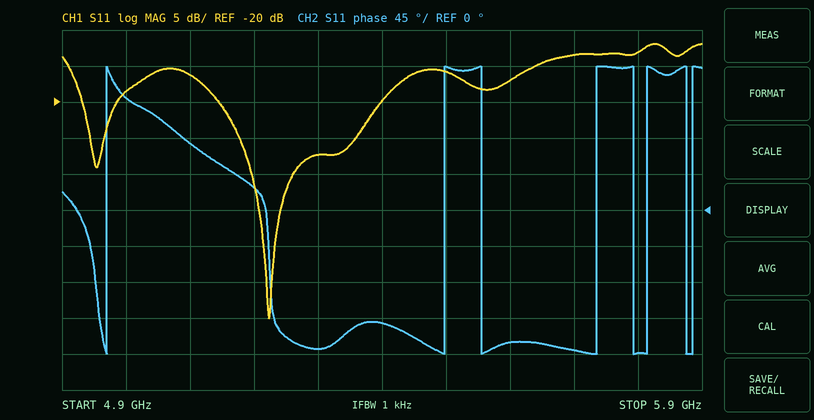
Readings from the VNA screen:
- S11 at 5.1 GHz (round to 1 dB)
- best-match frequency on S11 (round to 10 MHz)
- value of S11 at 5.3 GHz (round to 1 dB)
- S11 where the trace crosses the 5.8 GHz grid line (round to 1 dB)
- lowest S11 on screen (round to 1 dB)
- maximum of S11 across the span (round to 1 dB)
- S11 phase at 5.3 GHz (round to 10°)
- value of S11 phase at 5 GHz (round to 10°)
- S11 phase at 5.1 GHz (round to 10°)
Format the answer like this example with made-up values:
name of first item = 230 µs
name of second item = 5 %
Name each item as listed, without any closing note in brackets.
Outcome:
S11 at 5.1 GHz = -16 dB
best-match frequency on S11 = 5.22 GHz
value of S11 at 5.3 GHz = -27 dB
S11 where the trace crosses the 5.8 GHz grid line = -13 dB
lowest S11 on screen = -50 dB
maximum of S11 across the span = -12 dB
S11 phase at 5.3 GHz = -170°
value of S11 phase at 5 GHz = 140°
S11 phase at 5.1 GHz = 80°
